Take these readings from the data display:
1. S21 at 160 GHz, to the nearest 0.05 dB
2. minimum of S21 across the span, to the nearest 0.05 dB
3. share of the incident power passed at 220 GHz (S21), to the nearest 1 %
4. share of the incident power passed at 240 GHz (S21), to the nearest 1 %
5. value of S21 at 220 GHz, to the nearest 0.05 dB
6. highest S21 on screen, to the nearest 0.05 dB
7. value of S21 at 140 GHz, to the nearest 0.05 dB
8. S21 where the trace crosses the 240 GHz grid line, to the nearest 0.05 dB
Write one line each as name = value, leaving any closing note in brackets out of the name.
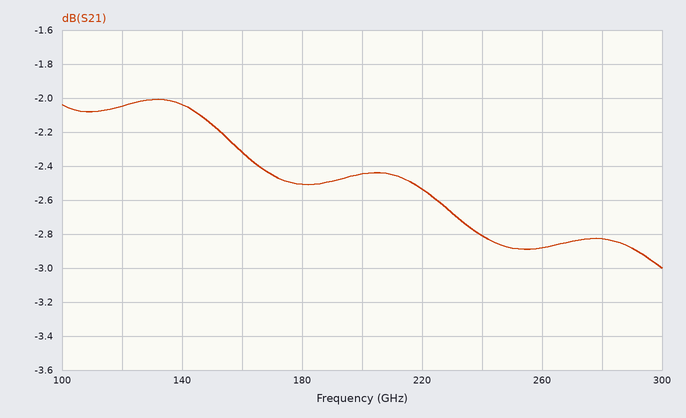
S21 at 160 GHz, to the nearest 0.05 dB = -2.30 dB
minimum of S21 across the span, to the nearest 0.05 dB = -3.00 dB
share of the incident power passed at 220 GHz (S21), to the nearest 1 % = 56 %
share of the incident power passed at 240 GHz (S21), to the nearest 1 % = 52 %
value of S21 at 220 GHz, to the nearest 0.05 dB = -2.55 dB
highest S21 on screen, to the nearest 0.05 dB = -2.00 dB
value of S21 at 140 GHz, to the nearest 0.05 dB = -2.05 dB
S21 where the trace crosses the 240 GHz grid line, to the nearest 0.05 dB = -2.80 dB
